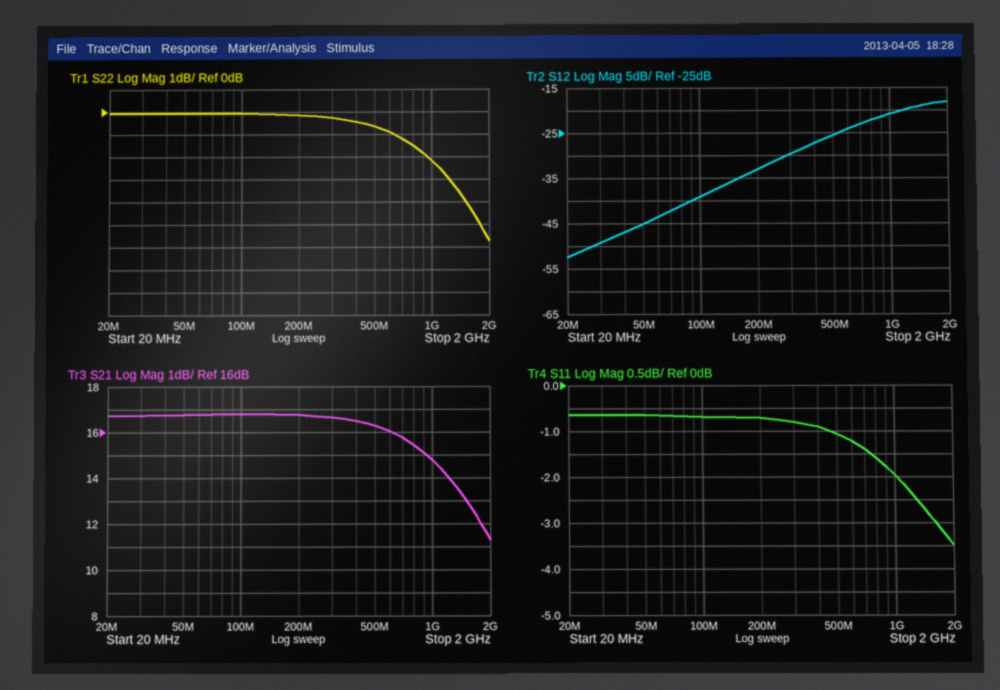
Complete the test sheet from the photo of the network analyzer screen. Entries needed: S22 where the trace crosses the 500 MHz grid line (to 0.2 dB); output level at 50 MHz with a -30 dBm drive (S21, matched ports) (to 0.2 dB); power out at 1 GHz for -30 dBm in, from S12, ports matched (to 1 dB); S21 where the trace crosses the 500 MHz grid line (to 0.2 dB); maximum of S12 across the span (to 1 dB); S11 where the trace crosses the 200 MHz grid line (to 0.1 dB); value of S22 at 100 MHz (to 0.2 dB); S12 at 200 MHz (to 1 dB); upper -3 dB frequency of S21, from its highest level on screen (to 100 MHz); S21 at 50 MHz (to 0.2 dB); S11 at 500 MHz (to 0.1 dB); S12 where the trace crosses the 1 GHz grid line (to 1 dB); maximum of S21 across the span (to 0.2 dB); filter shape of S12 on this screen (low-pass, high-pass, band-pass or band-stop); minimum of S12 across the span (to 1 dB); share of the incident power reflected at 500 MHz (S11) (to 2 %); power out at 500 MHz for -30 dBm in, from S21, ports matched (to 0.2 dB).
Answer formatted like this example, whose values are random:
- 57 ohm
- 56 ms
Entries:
- -0.6 dB
- -13.2 dBm
- -51 dBm
- 16.2 dB
- -18 dB
- -0.7 dB
- 0.0 dB
- -33 dB
- 1.3 GHz
- 16.8 dB
- -1.1 dB
- -21 dB
- 16.8 dB
- high-pass
- -52 dB
- 78 %
- -13.8 dBm
